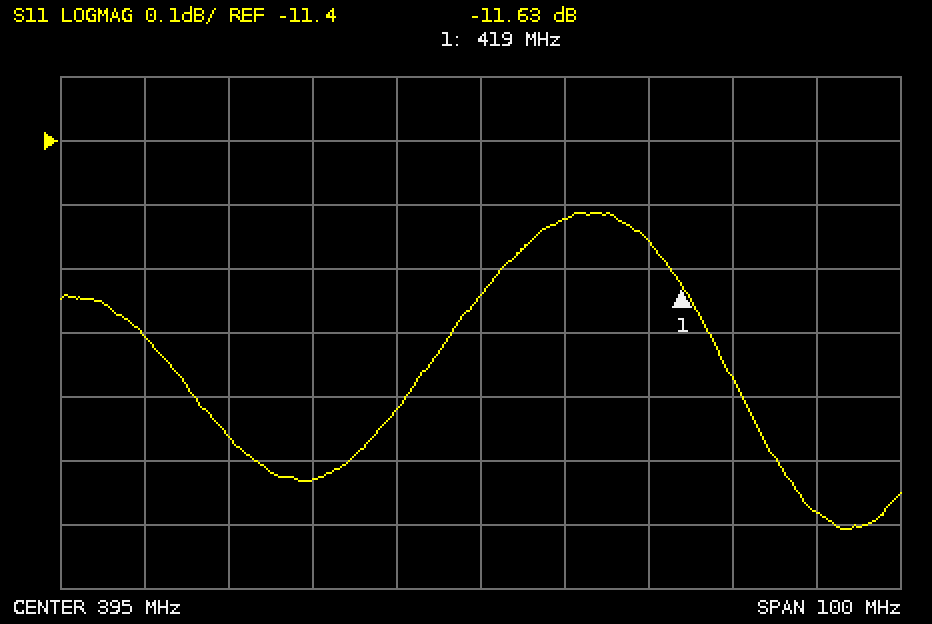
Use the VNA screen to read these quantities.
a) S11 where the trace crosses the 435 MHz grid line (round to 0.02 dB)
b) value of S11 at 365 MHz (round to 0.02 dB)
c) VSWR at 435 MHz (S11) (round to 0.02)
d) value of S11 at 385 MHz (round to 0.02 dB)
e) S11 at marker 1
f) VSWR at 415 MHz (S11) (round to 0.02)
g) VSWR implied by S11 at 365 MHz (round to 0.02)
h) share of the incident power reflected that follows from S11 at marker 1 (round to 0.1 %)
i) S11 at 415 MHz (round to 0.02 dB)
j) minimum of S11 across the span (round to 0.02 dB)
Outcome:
-11.98 dB
-11.86 dB
1.68
-11.82 dB
-11.63 dB
1.72
1.68
6.9 %
-11.56 dB
-12.00 dB
